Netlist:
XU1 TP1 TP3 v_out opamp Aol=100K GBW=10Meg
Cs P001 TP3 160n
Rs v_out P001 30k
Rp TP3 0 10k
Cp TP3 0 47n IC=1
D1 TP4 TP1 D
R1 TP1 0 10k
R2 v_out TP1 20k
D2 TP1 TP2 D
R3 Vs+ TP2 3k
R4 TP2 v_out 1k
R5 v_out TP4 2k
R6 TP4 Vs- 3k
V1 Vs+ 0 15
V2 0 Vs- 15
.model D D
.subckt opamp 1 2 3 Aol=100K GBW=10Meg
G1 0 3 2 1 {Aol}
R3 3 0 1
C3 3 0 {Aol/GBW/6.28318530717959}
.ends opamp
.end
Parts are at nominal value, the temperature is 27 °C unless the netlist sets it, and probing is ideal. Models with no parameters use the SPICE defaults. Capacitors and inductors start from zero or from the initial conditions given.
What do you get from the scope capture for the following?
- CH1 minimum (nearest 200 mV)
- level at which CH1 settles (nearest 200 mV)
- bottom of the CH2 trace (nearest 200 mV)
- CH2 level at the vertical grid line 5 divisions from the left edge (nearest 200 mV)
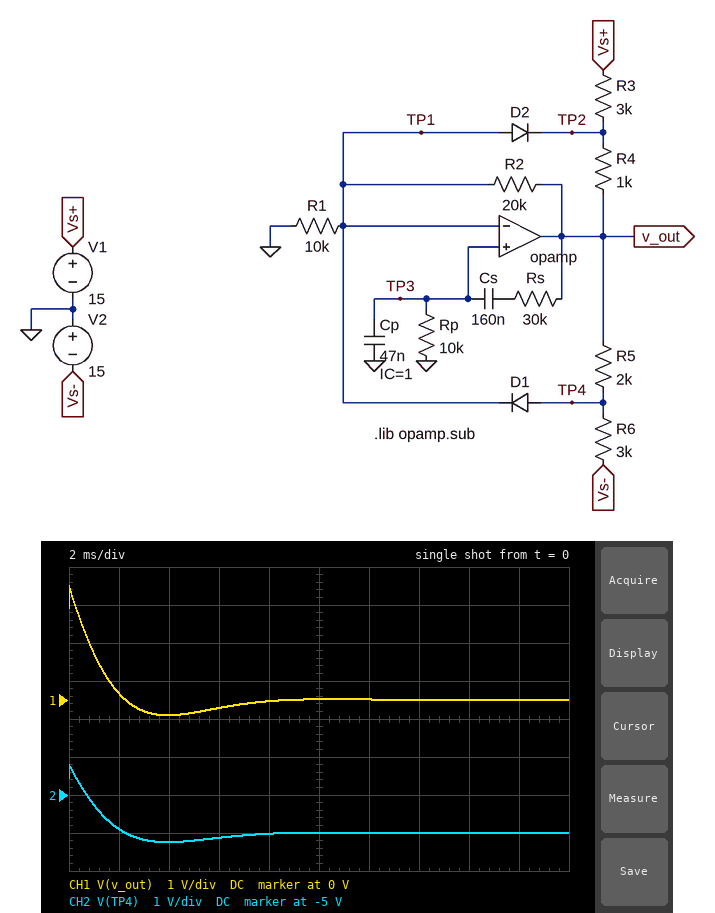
-400 mV
0 V
-6.2 V
-6.0 V
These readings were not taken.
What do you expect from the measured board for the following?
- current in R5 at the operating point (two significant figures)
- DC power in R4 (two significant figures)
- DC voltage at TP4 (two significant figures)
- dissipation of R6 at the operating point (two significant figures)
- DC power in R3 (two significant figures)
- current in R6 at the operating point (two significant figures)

3.0 mA
14 mW
-6.0 V
27 mW
42 mW
3.0 mA
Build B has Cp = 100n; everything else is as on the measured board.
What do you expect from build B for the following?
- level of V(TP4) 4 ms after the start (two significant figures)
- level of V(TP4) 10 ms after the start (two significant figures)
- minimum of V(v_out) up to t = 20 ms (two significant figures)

-6.0 V
-6.1 V
-440 mV
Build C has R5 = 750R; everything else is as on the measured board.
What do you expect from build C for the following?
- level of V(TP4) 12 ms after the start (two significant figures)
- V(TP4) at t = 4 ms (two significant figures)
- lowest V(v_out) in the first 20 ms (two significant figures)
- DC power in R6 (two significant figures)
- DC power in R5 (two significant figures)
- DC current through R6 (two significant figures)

-3.0 V
-3.3 V
-400 mV
48 mW
12 mW
4.0 mA
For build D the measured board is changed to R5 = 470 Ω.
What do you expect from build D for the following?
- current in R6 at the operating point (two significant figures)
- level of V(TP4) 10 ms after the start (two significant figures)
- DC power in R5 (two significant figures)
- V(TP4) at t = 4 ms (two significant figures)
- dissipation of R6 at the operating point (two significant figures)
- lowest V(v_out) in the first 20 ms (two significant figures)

4.3 mA
-2.0 V
8.8 mW
-2.4 V
56 mW
-400 mV
